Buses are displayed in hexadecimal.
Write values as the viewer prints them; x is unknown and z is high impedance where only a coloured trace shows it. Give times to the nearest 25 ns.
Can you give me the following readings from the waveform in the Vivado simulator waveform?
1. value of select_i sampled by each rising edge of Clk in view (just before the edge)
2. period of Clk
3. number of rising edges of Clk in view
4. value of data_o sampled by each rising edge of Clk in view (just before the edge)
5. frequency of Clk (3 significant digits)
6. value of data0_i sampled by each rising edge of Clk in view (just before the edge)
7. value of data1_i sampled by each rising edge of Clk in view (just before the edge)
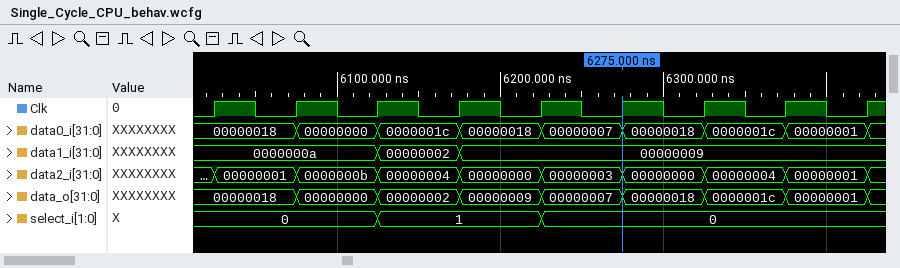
0, 0, 0, 1, 1, 0, 0, 0, 0
50 ns
9
00000018, 00000018, 00000000, 00000002, 00000009, 00000007, 00000018, 0000001c, 00000001
20.0 MHz
00000018, 00000018, 00000000, 0000001c, 00000018, 00000007, 00000018, 0000001c, 00000001
0000000a, 0000000a, 0000000a, 00000002, 00000009, 00000009, 00000009, 00000009, 00000009
